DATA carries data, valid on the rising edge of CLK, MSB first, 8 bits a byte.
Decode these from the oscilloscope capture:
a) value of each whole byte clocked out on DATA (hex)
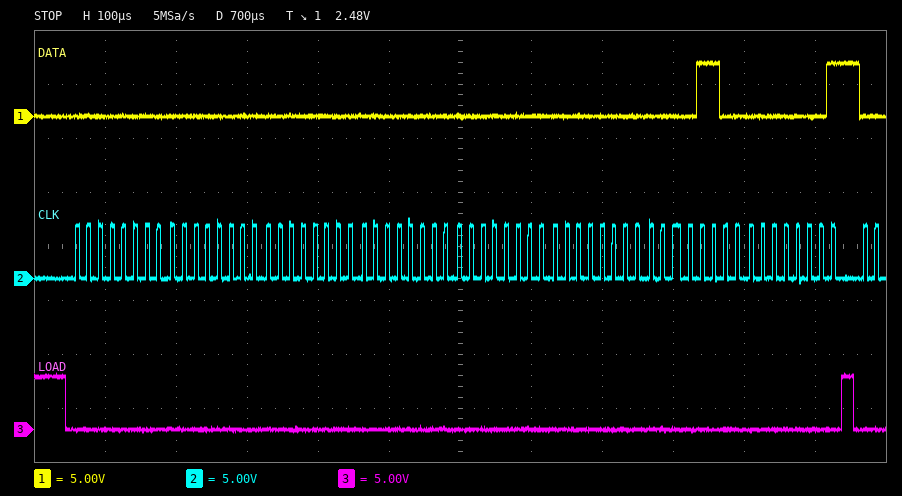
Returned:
00 00 00 00 00 00 0C 01
